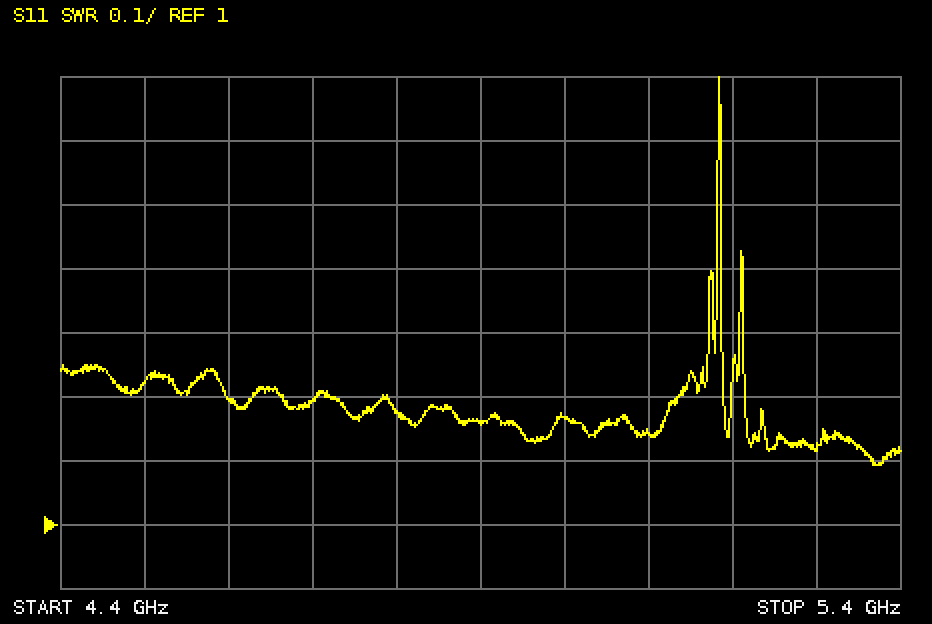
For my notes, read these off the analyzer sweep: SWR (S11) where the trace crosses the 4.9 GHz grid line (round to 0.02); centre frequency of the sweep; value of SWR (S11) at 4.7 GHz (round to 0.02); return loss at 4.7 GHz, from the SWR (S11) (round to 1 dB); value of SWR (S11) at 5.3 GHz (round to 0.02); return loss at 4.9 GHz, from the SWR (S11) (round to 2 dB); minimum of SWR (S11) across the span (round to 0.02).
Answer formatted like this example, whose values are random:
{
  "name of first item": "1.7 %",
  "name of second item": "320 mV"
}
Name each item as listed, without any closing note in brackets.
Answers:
{
  "SWR (S11) where the trace crosses the 4.9 GHz grid line": "1.16",
  "centre frequency of the sweep": "4.9 GHz",
  "value of SWR (S11) at 4.7 GHz": "1.20",
  "return loss at 4.7 GHz, from the SWR (S11)": "21 dB",
  "value of SWR (S11) at 5.3 GHz": "1.12",
  "return loss at 4.9 GHz, from the SWR (S11)": "22 dB",
  "minimum of SWR (S11) across the span": "1.10"
}
